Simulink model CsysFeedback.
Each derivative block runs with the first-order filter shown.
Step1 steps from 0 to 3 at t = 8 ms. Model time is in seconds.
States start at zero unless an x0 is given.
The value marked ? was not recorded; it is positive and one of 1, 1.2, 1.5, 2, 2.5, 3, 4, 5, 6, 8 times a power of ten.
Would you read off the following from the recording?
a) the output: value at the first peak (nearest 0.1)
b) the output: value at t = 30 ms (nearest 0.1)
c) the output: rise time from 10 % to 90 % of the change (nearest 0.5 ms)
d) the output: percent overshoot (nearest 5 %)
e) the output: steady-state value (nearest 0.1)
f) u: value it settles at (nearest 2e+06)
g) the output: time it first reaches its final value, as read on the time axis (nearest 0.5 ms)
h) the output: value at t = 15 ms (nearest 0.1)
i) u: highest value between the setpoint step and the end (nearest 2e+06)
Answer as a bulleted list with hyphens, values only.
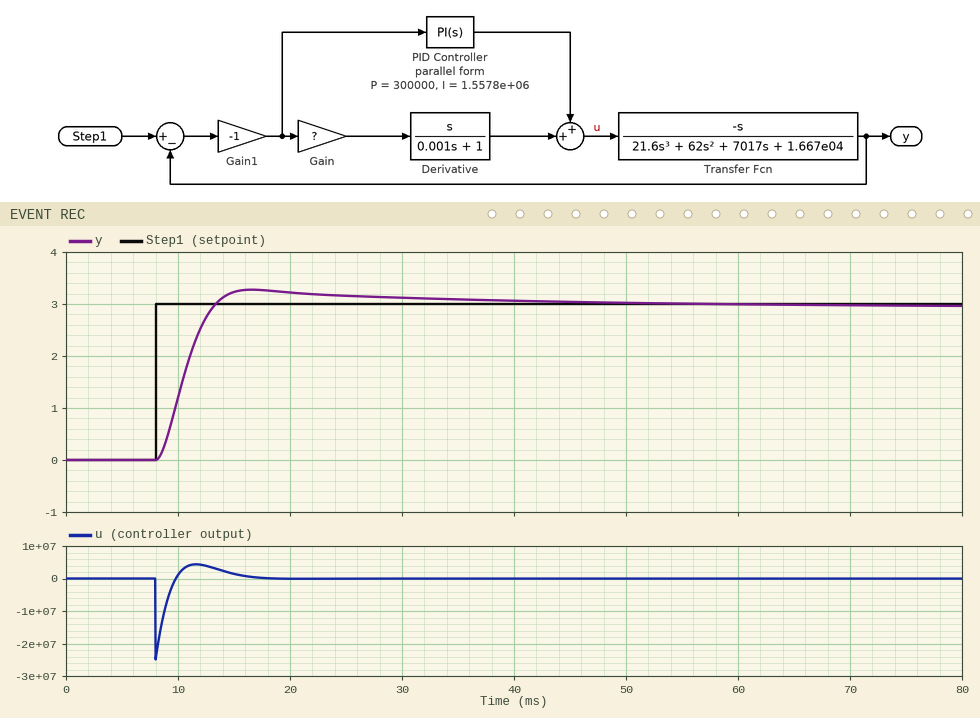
- 3.3
- 3.1
- 3.5 ms
- 10 %
- 3.0
- 0
- 13.0 ms
- 3.2
- 4000000
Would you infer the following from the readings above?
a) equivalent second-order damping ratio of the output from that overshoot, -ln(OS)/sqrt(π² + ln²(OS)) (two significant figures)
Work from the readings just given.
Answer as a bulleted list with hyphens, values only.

- 0.59
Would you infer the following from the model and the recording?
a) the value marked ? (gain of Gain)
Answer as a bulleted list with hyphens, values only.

- 8000
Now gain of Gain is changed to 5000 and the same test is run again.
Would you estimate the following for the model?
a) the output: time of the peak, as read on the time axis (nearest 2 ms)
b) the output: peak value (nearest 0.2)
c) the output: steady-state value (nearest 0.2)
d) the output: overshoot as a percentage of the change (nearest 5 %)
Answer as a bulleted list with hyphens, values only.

- 22 ms
- 3.4
- 3.0
- 15 %
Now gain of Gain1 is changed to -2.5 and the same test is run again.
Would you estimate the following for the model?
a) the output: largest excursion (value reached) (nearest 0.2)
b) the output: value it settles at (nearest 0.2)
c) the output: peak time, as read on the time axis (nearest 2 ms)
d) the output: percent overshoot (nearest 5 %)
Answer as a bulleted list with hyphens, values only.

- 3.6
- 3.0
- 12 ms
- 20 %
